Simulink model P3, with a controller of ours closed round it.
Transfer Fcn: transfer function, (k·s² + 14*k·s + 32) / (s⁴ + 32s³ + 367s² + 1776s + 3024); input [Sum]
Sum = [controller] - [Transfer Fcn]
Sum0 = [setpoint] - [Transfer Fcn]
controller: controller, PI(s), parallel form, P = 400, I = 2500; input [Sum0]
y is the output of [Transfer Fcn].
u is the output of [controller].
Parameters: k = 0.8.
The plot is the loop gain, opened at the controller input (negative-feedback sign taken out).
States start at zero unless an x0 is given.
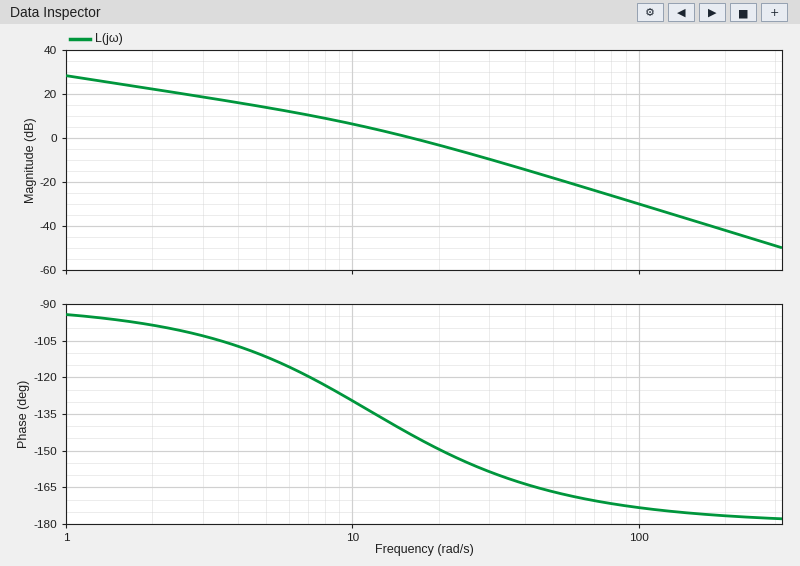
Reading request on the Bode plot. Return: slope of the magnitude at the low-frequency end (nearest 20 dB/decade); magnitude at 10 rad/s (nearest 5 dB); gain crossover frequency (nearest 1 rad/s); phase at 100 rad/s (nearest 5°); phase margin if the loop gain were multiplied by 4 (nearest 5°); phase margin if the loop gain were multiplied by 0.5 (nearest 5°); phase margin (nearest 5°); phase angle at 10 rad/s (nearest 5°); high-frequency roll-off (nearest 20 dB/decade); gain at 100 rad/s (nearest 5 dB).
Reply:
-20 dB/decade
5 dB
16 rad/s
-175°
20°
50°
35°
-130°
-40 dB/decade
-30 dB
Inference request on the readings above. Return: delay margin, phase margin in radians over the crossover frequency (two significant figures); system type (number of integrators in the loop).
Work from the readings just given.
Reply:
0.038 s
1
